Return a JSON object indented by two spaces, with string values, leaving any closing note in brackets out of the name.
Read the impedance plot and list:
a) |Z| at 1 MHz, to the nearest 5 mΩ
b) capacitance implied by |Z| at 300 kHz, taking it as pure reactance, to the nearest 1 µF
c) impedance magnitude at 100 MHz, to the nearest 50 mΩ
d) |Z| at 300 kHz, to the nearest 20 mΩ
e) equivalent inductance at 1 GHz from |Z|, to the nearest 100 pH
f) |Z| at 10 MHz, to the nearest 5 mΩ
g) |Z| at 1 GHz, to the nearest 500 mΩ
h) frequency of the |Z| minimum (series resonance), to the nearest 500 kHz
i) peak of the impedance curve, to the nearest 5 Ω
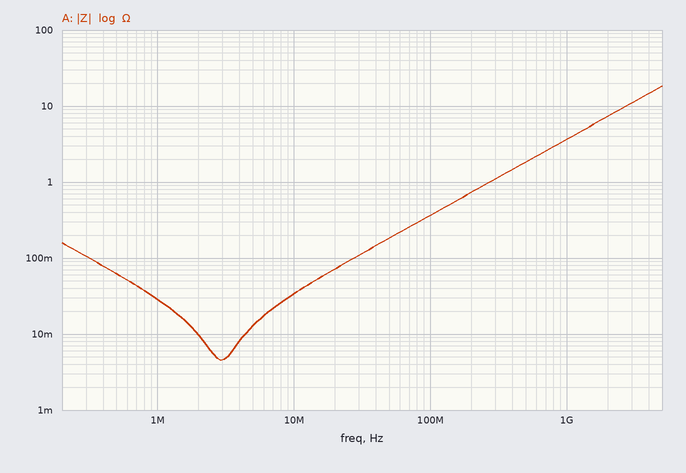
{
  "|Z| at 1 MHz, to the nearest 5 mΩ": "30 mΩ",
  "capacitance implied by |Z| at 300 kHz, taking it as pure reactance, to the nearest 1 µF": "5 µF",
  "impedance magnitude at 100 MHz, to the nearest 50 mΩ": "350 mΩ",
  "|Z| at 300 kHz, to the nearest 20 mΩ": "100 mΩ",
  "equivalent inductance at 1 GHz from |Z|, to the nearest 100 pH": "600 pH",
  "|Z| at 10 MHz, to the nearest 5 mΩ": "35 mΩ",
  "|Z| at 1 GHz, to the nearest 500 mΩ": "3.5 Ω",
  "frequency of the |Z| minimum (series resonance), to the nearest 500 kHz": "3.0 MHz",
  "peak of the impedance curve, to the nearest 5 Ω": "20 Ω"
}
